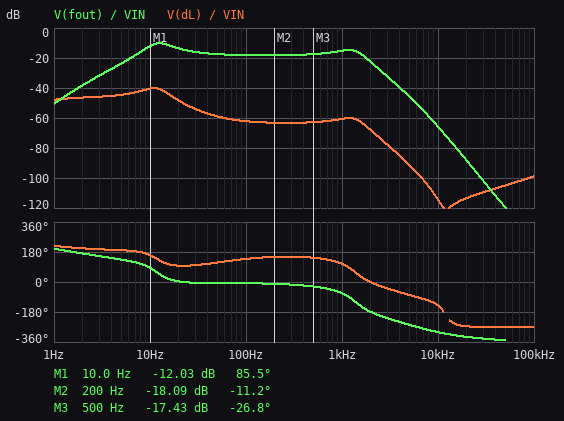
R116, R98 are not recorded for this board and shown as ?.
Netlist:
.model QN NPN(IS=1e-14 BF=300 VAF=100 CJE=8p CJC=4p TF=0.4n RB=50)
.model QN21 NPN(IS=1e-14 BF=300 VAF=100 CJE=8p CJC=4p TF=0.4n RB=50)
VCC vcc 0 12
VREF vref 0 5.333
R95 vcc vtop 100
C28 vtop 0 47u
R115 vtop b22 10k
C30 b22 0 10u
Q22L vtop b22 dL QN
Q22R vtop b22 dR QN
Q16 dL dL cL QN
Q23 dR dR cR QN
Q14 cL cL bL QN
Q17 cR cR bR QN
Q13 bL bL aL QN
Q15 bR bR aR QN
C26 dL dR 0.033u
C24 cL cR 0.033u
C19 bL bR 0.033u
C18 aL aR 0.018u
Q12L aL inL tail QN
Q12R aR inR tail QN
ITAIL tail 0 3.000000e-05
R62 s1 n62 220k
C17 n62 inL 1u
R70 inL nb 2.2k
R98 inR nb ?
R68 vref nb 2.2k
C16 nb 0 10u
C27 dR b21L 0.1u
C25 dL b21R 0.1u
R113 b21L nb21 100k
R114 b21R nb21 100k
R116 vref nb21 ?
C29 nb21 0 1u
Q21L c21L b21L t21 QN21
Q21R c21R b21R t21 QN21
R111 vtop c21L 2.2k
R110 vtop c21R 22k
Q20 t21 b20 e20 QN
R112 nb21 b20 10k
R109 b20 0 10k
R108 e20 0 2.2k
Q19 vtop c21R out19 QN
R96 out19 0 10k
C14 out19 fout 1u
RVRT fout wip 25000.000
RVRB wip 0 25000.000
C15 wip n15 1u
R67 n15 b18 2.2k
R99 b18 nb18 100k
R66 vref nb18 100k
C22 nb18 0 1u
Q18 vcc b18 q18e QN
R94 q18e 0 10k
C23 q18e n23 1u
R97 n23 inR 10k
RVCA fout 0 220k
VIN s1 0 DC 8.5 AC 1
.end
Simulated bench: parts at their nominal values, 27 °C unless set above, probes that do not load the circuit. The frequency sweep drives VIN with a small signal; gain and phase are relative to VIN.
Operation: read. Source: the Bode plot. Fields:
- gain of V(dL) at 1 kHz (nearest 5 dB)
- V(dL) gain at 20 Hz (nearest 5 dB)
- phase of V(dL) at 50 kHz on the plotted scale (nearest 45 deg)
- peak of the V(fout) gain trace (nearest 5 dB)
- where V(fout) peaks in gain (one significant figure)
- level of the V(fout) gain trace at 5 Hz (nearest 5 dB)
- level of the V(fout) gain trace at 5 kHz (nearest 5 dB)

-60 dB
-50 dB
-270 deg
-10 dB
10 Hz
-25 dB
-45 dB
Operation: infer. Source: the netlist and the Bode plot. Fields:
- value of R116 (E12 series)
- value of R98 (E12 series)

12 kΩ
1.8 kΩ
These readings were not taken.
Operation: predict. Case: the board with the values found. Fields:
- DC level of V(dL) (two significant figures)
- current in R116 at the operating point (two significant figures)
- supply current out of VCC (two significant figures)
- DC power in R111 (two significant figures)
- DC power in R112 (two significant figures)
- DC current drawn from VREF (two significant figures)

11 V
170 µA
1.6 mA
120 µW
280 µW
170 µA
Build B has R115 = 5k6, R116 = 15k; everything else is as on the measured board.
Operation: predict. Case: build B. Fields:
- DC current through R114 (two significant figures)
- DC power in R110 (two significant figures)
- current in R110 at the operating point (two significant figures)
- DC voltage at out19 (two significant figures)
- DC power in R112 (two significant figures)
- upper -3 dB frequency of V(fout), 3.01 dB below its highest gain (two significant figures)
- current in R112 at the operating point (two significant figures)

620 nA
850 µW
200 µA
6.9 V
230 µW
20 Hz
150 µA
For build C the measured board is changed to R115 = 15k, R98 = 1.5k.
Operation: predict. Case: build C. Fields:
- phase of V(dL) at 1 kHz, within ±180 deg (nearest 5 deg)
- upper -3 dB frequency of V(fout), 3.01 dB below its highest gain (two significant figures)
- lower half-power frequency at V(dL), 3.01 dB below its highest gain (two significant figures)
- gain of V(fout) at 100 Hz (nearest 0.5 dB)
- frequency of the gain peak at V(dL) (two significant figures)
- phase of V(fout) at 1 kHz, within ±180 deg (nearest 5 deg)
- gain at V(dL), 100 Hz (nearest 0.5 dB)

100 deg
22 Hz
6.3 Hz
-17.0 dB
12 Hz
-75 deg
-61.0 dB
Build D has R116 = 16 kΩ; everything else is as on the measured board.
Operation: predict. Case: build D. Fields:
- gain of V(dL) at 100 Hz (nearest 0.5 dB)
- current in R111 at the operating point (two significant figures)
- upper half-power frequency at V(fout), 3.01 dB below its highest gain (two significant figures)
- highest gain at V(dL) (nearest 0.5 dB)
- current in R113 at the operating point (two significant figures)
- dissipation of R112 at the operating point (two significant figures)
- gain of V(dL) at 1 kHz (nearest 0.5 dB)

-61.0 dB
190 µA
20 Hz
-40.5 dB
590 nA
220 µW
-60.0 dB
